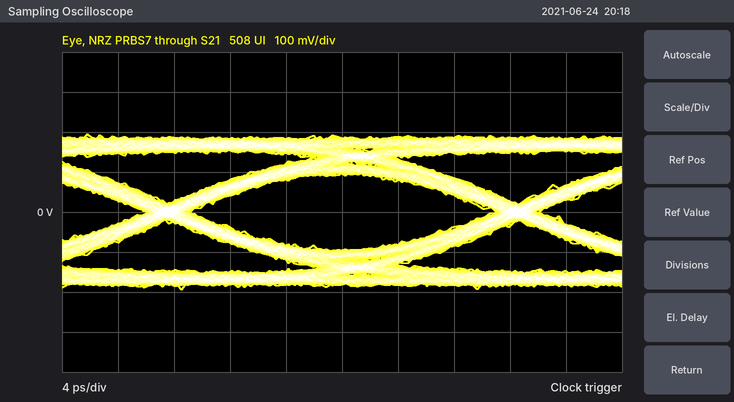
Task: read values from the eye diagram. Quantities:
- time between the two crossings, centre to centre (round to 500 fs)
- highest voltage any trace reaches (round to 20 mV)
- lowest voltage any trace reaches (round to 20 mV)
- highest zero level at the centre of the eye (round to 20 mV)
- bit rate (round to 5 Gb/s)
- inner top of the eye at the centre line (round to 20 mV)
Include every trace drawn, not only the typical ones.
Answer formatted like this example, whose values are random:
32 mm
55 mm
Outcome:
25.0 ps
200 mV
-200 mV
-100 mV
40 Gb/s
100 mV
